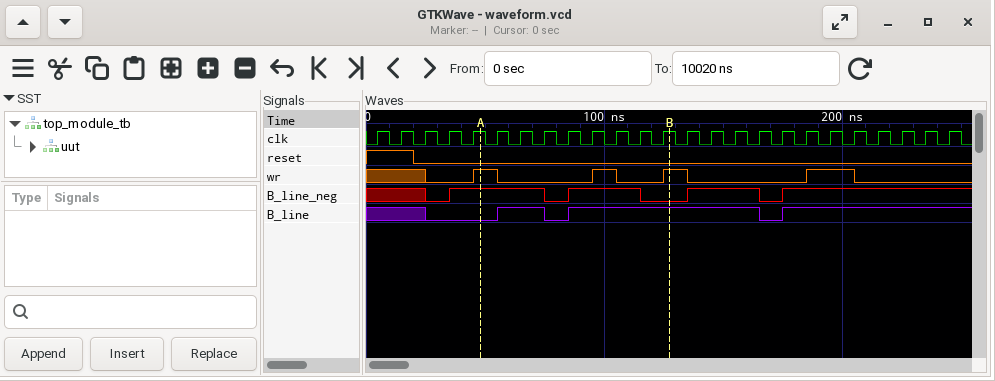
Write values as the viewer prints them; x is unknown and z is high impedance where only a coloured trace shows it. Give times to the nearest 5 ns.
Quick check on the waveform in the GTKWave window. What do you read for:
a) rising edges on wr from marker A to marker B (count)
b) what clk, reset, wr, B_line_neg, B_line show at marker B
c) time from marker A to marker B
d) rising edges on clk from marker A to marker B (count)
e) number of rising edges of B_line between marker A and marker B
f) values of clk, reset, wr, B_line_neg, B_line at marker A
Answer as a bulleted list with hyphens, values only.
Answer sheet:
- 2
- clk=1, reset=0, wr=1, B_line_neg=0, B_line=1
- 80 ns
- 8
- 2
- clk=1, reset=0, wr=1, B_line_neg=1, B_line=0
